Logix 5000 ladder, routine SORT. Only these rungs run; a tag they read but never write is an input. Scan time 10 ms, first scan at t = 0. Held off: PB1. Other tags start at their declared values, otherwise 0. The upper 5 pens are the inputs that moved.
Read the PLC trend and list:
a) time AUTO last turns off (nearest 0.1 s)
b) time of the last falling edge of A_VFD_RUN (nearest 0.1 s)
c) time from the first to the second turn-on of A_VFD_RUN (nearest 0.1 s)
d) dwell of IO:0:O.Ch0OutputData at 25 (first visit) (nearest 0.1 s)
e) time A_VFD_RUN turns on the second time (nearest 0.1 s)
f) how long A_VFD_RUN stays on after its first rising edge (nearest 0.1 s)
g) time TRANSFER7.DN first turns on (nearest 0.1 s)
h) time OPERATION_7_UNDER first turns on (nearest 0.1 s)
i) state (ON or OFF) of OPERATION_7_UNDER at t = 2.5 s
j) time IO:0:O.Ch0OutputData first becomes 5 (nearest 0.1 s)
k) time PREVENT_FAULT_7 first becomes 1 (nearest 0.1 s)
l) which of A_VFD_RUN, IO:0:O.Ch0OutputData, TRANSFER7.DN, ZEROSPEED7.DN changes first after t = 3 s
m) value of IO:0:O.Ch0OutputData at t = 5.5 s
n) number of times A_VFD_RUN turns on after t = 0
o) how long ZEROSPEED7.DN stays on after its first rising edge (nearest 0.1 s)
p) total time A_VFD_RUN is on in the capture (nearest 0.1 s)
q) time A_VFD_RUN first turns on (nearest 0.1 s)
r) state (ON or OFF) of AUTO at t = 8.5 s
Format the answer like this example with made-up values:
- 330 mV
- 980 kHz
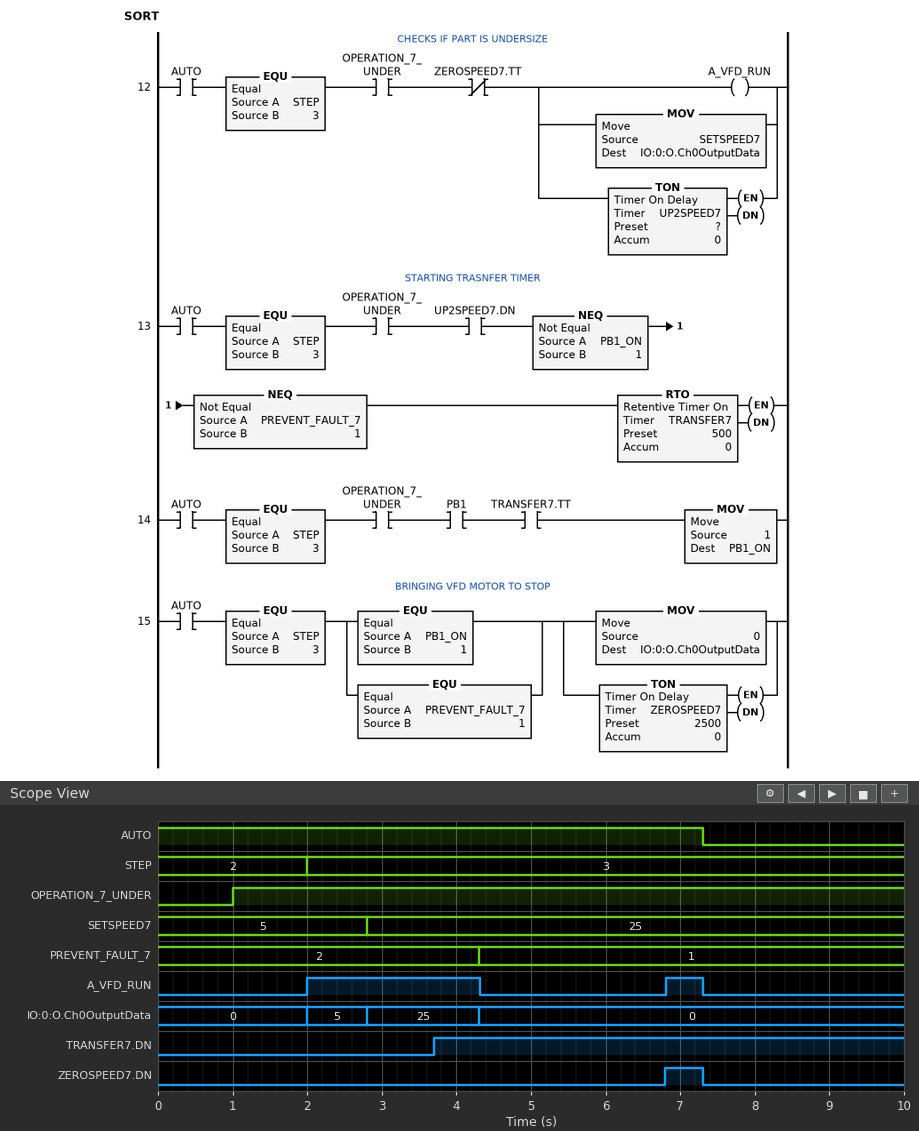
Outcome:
- 7.3 s
- 7.3 s
- 4.8 s
- 1.5 s
- 6.8 s
- 2.3 s
- 3.7 s
- 1.0 s
- ON
- 2.0 s
- 4.3 s
- TRANSFER7.DN
- 0
- 2
- 0.5 s
- 2.8 s
- 2.0 s
- OFF
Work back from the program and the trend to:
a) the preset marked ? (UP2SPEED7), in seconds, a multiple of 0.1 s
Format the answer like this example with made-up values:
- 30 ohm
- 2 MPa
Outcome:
- 1.2 s
